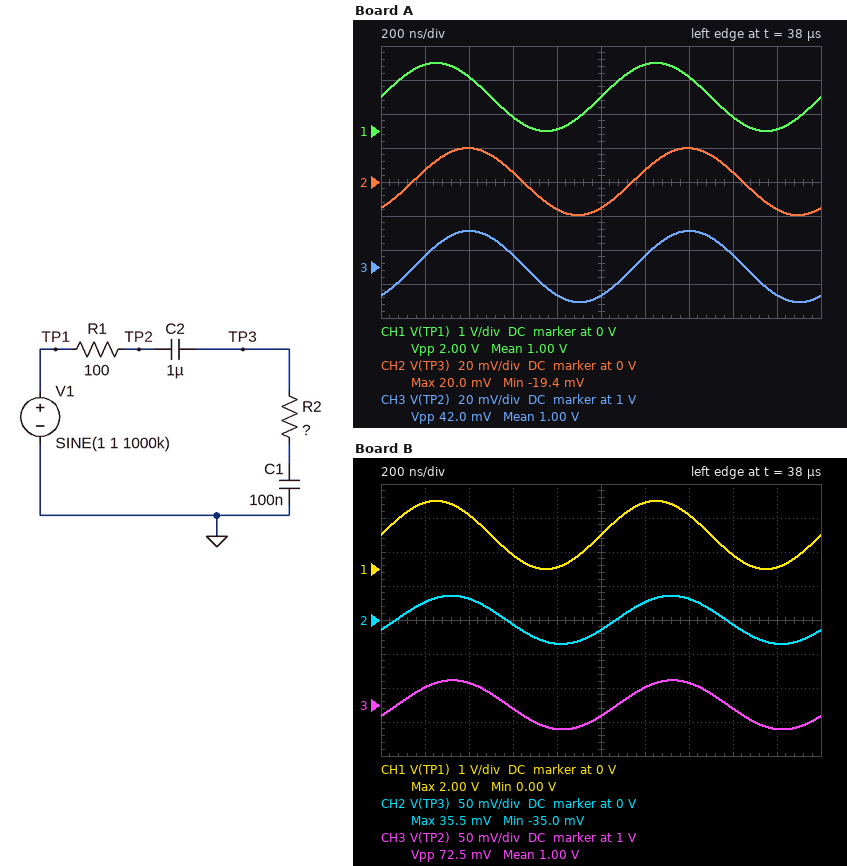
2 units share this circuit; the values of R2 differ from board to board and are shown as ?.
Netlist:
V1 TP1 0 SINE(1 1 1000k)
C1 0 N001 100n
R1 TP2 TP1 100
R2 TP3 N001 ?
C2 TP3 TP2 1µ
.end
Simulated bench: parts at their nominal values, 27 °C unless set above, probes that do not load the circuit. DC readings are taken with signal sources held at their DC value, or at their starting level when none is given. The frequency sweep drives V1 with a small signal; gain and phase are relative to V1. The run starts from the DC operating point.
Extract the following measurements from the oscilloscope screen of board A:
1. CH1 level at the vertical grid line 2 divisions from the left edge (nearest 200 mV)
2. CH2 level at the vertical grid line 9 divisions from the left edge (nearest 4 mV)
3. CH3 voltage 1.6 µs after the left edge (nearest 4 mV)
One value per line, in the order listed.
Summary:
1.6 V
-16 mV
1.008 V
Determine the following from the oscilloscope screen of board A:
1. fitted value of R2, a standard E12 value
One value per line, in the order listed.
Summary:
1.2 Ω
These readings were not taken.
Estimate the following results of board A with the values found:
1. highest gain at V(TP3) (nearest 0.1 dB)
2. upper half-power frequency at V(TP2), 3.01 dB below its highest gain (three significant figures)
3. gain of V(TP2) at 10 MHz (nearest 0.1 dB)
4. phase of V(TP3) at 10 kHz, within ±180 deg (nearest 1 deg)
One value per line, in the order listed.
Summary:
-0.8 dB
17.3 kHz
-38.4 dB
-30 deg
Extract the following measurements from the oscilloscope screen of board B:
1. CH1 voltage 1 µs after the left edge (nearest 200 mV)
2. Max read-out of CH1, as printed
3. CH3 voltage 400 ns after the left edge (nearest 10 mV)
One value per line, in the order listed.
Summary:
1.0 V
2.00 V
1.03 V
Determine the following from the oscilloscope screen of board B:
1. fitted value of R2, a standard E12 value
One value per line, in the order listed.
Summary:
3.3 Ω
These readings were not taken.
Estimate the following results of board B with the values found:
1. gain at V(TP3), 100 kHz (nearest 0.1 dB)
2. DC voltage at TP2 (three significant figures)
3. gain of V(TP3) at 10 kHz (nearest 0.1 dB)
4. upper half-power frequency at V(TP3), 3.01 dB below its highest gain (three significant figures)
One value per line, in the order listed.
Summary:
-16.2 dB
1.00 V
-2.1 dB
17.0 kHz
